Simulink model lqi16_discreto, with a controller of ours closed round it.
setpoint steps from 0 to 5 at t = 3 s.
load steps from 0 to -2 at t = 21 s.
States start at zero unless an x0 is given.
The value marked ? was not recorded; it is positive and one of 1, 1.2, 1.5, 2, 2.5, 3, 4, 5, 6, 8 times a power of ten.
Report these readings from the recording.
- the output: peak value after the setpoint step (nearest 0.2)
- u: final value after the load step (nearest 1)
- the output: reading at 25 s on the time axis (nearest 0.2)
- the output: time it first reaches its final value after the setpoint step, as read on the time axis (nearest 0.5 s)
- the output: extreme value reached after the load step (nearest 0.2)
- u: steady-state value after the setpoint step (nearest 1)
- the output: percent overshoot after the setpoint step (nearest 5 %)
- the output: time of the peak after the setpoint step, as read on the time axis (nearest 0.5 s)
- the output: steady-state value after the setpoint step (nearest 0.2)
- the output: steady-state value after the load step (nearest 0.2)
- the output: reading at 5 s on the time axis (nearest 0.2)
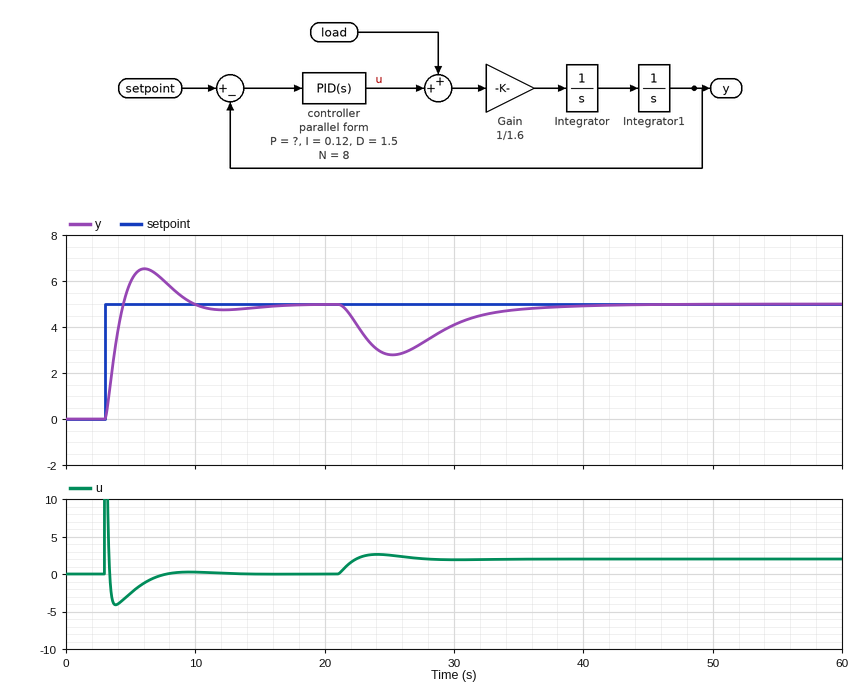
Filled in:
6.6
2
2.8
4.5 s
2.8
0
30 %
6.0 s
5.0
5.0
6.0
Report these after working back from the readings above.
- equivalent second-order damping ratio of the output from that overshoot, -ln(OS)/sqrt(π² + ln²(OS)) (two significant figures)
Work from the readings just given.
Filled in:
0.36
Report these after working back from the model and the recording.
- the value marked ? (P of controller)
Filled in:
0.8
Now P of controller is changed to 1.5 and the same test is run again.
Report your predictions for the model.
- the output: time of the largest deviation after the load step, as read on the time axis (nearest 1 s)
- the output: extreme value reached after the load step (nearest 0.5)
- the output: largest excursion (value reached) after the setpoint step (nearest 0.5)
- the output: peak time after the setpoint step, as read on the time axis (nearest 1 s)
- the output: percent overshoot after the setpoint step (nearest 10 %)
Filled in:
24 s
3.5
7.0
5 s
40 %
